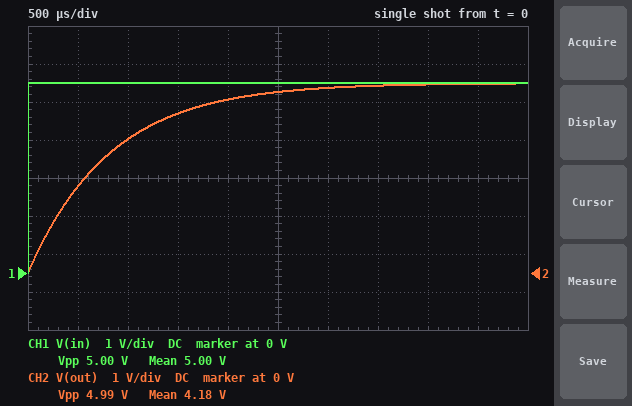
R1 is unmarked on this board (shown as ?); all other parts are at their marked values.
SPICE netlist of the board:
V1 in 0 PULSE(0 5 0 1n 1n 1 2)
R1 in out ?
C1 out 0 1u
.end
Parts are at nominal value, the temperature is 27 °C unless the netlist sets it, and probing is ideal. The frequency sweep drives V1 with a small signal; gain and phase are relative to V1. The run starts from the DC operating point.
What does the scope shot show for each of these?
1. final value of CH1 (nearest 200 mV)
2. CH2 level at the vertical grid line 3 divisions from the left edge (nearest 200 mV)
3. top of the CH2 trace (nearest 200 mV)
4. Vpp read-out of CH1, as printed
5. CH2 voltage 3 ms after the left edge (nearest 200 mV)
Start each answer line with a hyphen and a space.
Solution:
- 5.0 V
- 4.2 V
- 5.0 V
- 5.00 V
- 4.8 V
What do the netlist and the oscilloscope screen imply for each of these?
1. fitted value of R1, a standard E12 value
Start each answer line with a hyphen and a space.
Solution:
- 820 Ω
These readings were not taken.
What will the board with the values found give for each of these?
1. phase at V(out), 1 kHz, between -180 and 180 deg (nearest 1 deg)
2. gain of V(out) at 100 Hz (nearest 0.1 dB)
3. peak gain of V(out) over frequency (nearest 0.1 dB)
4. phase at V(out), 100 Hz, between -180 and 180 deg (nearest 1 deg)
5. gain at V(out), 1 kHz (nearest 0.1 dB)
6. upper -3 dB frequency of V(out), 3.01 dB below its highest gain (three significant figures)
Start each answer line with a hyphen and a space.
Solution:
- -79 deg
- -1.0 dB
- 0 dB
- -27 deg
- -14.4 dB
- 194 Hz
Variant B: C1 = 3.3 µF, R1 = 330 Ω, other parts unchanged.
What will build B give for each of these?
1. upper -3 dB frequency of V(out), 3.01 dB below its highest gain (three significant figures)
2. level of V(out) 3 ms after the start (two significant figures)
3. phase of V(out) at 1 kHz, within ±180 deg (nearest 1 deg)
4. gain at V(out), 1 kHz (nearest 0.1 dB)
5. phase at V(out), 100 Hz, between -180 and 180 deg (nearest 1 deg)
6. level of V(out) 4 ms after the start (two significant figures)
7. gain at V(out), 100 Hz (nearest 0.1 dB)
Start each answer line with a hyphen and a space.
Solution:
- 146 Hz
- 4.7 V
- -82 deg
- -16.8 dB
- -34 deg
- 4.9 V
- -1.7 dB
